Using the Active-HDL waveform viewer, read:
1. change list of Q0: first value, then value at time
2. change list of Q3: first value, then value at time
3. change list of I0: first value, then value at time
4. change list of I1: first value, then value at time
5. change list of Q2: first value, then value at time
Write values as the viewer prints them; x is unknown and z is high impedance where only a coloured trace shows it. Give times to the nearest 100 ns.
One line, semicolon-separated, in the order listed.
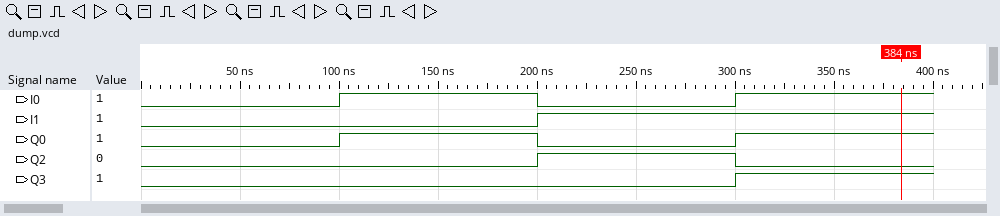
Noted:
0, 1 at 100 ns, 0 at 200 ns, 1 at 300 ns; 0, 1 at 300 ns; 0, 1 at 100 ns, 0 at 200 ns, 1 at 300 ns; 0, 1 at 200 ns; 0, 1 at 200 ns, 0 at 300 ns
